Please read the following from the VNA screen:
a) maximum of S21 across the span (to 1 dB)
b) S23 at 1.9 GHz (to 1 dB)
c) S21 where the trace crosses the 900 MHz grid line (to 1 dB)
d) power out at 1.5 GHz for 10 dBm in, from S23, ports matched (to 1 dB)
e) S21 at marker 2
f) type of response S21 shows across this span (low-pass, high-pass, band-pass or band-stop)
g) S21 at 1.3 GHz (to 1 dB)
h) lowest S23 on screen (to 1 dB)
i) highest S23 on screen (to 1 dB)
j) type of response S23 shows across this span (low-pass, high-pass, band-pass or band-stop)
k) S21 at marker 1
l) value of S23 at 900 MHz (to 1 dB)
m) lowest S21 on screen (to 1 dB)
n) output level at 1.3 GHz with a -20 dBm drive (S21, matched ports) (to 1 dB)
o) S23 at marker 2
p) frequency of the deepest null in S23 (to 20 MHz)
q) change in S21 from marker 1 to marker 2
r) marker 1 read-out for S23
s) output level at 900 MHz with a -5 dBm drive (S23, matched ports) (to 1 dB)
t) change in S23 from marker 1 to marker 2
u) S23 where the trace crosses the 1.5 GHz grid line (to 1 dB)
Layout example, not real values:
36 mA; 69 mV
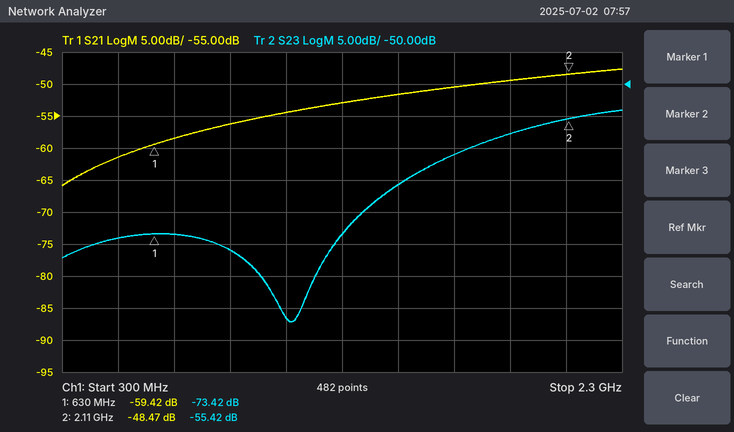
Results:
-48 dB; -58 dB; -56 dB; -56 dBm; -48.47 dB; high-pass; -53 dB; -87 dB; -54 dB; high-pass; -59.42 dB; -76 dB; -66 dB; -73 dBm; -55.42 dB; 1.12 GHz; 10.95 dB; -73.42 dB; -81 dBm; 18.00 dB; -66 dB
